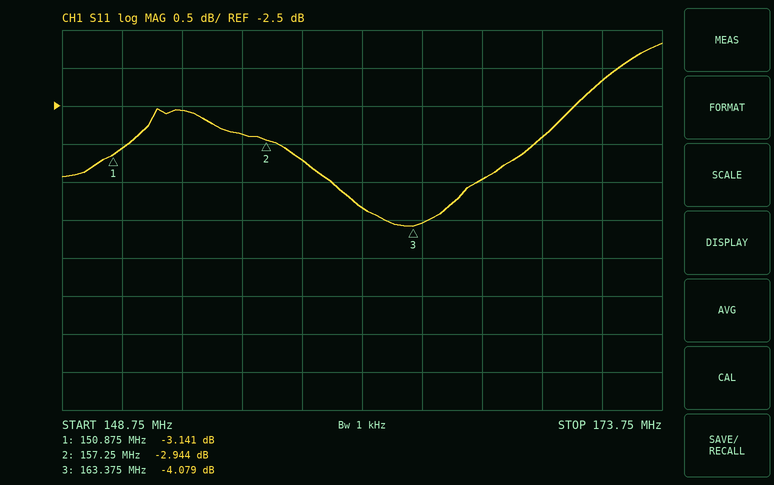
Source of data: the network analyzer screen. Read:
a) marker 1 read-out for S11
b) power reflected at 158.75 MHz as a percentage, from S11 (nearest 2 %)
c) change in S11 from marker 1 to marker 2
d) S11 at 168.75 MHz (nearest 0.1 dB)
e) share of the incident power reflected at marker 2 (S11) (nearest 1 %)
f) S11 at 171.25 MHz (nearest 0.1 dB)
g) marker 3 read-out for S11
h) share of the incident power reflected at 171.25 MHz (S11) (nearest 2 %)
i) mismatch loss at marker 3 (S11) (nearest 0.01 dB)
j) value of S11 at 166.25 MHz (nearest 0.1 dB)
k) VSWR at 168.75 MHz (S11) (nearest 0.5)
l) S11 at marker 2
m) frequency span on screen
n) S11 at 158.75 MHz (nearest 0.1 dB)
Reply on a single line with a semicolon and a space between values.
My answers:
-3.141 dB; 48 %; 0.197 dB; -2.9 dB; 51 %; -2.2 dB; -4.079 dB; 60 %; 2.15 dB; -3.5 dB; 6.0; -2.944 dB; 25 MHz; -3.2 dB
